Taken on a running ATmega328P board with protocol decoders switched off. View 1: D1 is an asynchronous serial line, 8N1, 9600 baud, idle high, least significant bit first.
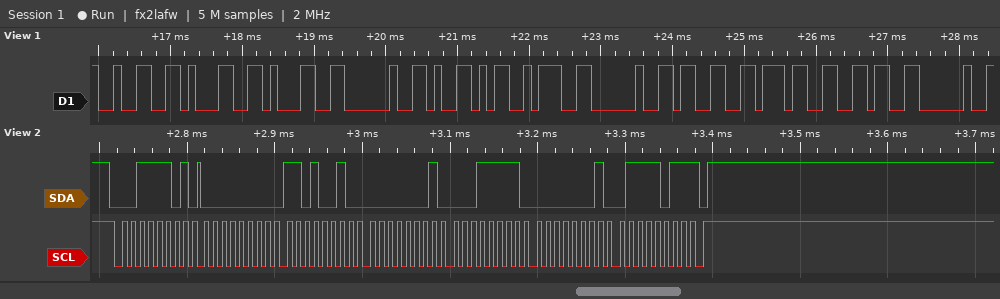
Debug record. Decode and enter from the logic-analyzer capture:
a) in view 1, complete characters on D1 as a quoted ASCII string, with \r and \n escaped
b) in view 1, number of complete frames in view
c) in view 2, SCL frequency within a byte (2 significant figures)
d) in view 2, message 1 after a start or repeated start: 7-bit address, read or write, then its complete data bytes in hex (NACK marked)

"211 Y: 376 "
11
100 kHz
0x1E read: 00 D2 01 1F 01 7B NACK
